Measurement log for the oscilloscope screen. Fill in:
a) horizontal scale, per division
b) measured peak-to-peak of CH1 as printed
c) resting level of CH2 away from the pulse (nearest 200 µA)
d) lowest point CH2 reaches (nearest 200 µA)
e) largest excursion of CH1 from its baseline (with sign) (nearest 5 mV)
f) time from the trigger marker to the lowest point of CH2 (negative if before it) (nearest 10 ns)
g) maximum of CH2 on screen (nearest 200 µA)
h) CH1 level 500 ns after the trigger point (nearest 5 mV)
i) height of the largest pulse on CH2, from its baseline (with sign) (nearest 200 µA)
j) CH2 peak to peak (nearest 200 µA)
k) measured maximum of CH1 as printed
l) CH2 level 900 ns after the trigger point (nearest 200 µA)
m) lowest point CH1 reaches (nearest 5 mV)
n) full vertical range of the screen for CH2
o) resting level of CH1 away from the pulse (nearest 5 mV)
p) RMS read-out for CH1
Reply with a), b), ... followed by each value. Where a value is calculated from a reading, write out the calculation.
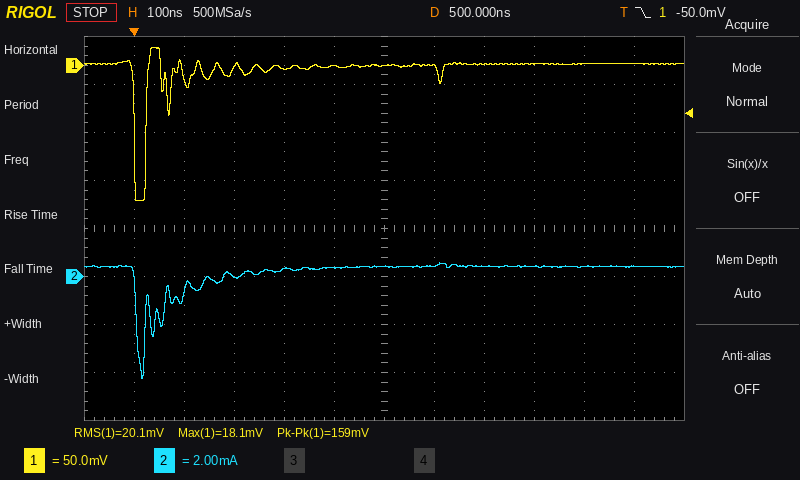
a) 100 ns
b) 159 mV
c) 400 µA
d) -4.2 mA
e) -140 mV − (0 mV) = -140 mV
f) +20 ns
g) 600 µA
h) 0 mV
i) -4.2 mA − (400 µA) = -4.6 mA
j) 600 µA − (-4.2 mA) = 4.8 mA
k) 18.1 mV
l) 400 µA
m) -140 mV
n) 16 mA
o) 0 mV
p) 20.1 mV
